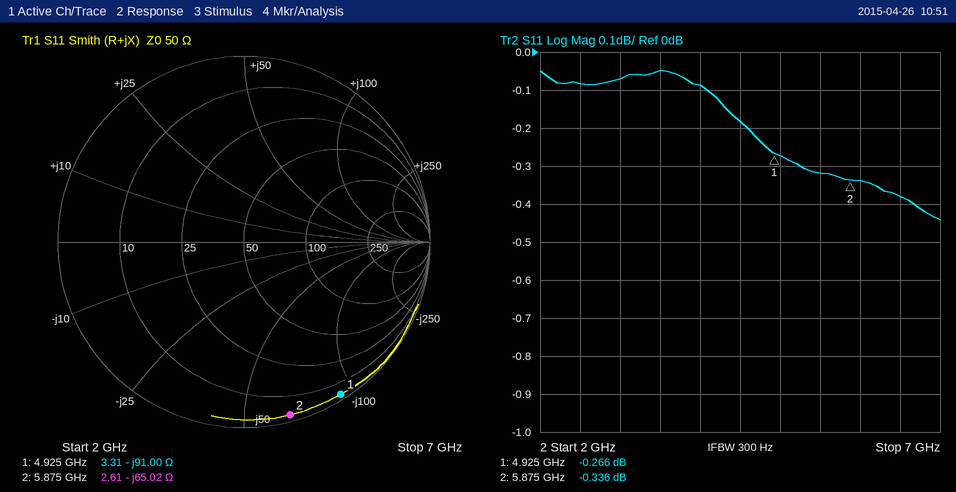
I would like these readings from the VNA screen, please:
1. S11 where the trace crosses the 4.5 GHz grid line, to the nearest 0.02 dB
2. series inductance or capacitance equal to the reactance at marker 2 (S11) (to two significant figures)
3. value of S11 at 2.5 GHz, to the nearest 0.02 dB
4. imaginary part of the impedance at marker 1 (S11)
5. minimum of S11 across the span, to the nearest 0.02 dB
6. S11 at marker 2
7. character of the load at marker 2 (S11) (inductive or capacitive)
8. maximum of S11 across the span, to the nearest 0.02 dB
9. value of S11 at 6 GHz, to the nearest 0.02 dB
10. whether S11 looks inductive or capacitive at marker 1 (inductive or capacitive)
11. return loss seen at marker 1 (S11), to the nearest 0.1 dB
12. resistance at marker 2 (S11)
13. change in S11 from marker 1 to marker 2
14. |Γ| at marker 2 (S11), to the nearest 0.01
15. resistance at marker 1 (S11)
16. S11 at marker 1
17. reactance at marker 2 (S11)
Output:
-0.18 dB
420 fF
-0.08 dB
-91.00 Ω
-0.44 dB
-0.336 dB
capacitive
-0.04 dB
-0.34 dB
capacitive
0.3 dB
2.61 Ω
-0.070 dB
0.96
3.31 Ω
-0.266 dB
-65.02 Ω
